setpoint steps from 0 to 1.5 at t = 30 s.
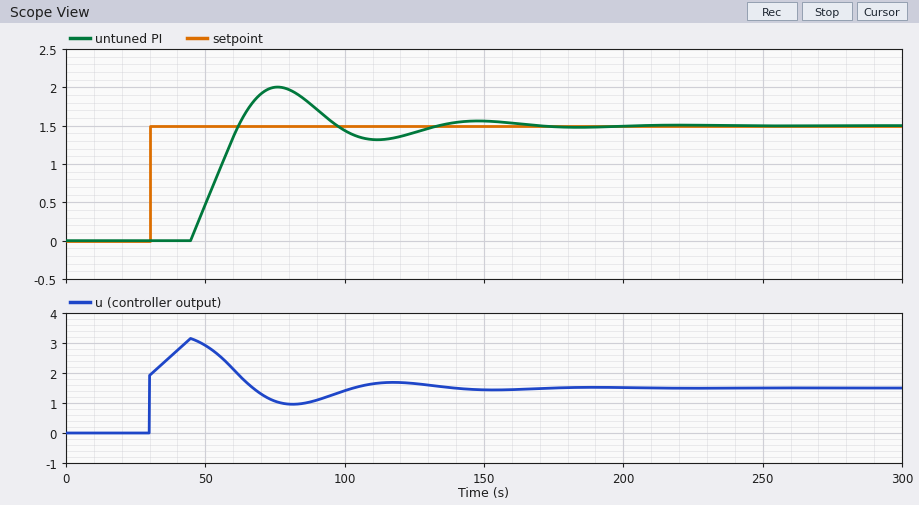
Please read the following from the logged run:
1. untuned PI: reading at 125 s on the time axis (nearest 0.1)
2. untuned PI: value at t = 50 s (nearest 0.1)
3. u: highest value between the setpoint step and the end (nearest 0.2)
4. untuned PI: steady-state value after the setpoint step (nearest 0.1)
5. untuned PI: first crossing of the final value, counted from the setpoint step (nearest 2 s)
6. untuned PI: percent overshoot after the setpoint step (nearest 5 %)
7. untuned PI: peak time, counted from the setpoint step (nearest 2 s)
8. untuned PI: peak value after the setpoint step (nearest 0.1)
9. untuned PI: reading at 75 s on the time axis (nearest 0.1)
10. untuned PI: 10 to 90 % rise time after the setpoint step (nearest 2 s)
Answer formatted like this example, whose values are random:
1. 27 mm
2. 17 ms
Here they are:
1. 1.4
2. 0.5
3. 3.2
4. 1.5
5. 32 s
6. 35 %
7. 46 s
8. 2.0
9. 2.0
10. 14 s
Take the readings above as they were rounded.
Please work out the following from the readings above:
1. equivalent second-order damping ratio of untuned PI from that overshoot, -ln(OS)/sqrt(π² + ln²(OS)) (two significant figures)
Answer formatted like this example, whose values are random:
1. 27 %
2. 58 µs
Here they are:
1. 0.32
